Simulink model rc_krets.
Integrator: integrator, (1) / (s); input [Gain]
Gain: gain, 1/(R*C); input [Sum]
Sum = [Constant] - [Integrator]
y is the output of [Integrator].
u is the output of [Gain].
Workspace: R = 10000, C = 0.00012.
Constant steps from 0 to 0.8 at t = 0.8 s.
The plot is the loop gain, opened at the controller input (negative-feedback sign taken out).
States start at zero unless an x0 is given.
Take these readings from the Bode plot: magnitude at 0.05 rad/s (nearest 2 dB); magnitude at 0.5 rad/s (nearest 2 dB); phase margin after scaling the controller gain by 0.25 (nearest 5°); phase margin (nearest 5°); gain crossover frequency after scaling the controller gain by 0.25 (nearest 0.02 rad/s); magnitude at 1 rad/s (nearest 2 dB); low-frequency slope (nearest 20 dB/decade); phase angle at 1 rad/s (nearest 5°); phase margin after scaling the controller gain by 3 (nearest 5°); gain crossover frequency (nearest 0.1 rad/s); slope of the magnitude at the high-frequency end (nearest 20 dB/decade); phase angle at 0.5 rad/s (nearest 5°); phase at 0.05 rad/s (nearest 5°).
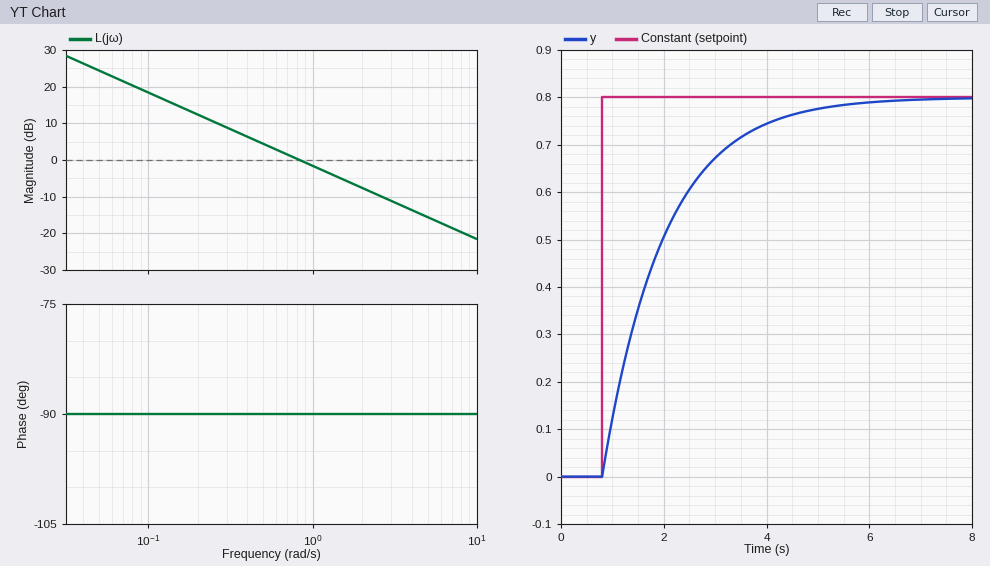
24 dB
4 dB
90°
90°
0.20 rad/s
-2 dB
-20 dB/decade
-90°
90°
0.8 rad/s
-20 dB/decade
-90°
-90°
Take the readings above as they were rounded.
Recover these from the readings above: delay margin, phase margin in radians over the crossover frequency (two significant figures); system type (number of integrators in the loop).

2.0 s
1
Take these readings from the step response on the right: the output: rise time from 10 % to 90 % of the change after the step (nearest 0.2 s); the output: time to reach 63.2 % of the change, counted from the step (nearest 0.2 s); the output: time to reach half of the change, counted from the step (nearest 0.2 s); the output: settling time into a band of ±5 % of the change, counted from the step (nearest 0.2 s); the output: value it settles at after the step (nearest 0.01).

2.6 s
1.2 s
0.8 s
3.6 s
0.80
